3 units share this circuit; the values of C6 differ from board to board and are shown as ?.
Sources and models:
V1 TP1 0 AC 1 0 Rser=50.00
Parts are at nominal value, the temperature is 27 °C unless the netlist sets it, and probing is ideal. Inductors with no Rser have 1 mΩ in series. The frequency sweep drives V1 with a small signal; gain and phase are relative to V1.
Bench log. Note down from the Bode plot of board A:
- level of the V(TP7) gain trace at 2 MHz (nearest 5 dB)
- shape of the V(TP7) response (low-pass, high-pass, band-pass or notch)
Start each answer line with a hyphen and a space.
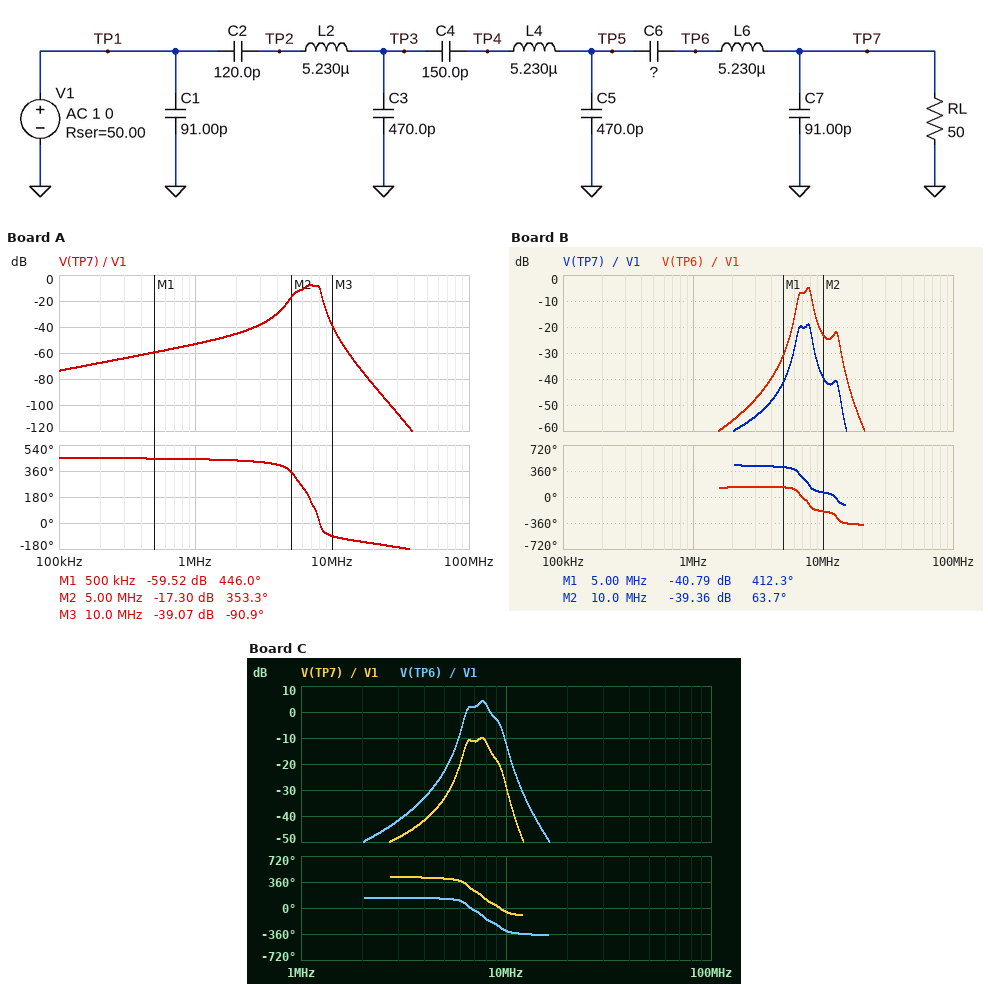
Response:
- -45 dB
- band-pass
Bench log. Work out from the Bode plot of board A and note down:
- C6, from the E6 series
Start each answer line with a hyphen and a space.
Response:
- 220 pF
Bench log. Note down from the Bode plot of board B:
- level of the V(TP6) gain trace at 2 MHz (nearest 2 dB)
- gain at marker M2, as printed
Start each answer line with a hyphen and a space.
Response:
- -56 dB
- -39.36 dB
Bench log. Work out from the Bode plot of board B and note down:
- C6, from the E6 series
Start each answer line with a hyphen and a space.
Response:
- 33 pF
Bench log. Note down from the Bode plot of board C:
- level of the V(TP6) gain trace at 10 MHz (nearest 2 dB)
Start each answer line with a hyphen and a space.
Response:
- -12 dB
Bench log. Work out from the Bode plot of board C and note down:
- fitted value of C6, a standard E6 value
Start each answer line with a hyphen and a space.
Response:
- 68 pF
